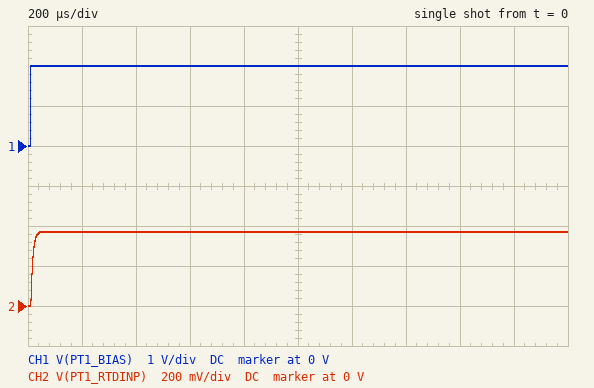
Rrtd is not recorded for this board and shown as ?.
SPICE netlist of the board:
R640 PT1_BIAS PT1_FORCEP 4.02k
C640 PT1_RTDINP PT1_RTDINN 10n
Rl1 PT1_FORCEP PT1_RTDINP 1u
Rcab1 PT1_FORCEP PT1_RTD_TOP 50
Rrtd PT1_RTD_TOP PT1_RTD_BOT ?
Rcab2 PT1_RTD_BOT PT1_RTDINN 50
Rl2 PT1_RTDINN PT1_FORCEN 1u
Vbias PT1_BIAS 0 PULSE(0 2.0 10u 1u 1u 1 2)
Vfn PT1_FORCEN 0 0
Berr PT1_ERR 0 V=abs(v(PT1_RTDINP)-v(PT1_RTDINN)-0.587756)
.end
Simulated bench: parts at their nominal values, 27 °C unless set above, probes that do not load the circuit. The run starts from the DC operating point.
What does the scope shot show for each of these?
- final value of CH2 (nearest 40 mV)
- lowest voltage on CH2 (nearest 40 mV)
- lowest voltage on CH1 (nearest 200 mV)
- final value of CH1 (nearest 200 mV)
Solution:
360 mV
0 V
0 V
2.0 V
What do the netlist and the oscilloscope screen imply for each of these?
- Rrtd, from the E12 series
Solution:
820 Ω
